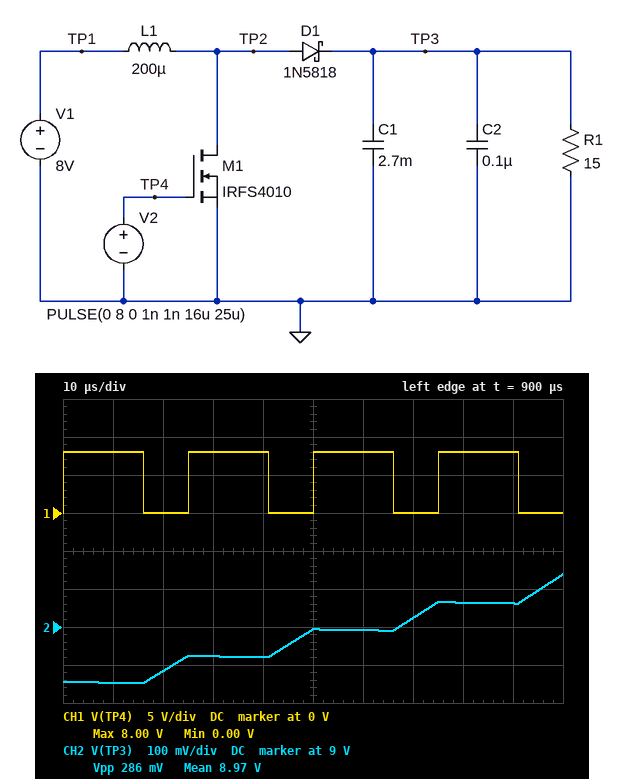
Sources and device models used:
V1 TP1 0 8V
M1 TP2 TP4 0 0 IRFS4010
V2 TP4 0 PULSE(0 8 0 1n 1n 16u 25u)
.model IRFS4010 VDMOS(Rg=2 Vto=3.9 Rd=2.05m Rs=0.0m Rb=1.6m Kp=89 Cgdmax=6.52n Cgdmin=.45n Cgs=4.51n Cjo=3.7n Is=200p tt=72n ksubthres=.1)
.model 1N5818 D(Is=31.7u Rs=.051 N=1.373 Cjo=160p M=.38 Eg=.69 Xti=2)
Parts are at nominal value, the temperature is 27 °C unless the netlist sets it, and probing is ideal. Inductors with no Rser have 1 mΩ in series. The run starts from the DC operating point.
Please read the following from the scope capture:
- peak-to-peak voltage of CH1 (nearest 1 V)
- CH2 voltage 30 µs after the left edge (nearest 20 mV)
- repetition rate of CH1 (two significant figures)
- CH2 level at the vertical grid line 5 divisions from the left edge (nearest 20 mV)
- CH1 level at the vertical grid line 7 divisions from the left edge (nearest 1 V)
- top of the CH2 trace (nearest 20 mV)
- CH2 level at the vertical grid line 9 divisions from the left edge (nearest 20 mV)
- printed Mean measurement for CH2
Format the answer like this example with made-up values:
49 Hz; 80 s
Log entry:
8 V; 8.92 V; 40 kHz; 9.00 V; 0 V; 9.14 V; 9.06 V; 8.97 V
